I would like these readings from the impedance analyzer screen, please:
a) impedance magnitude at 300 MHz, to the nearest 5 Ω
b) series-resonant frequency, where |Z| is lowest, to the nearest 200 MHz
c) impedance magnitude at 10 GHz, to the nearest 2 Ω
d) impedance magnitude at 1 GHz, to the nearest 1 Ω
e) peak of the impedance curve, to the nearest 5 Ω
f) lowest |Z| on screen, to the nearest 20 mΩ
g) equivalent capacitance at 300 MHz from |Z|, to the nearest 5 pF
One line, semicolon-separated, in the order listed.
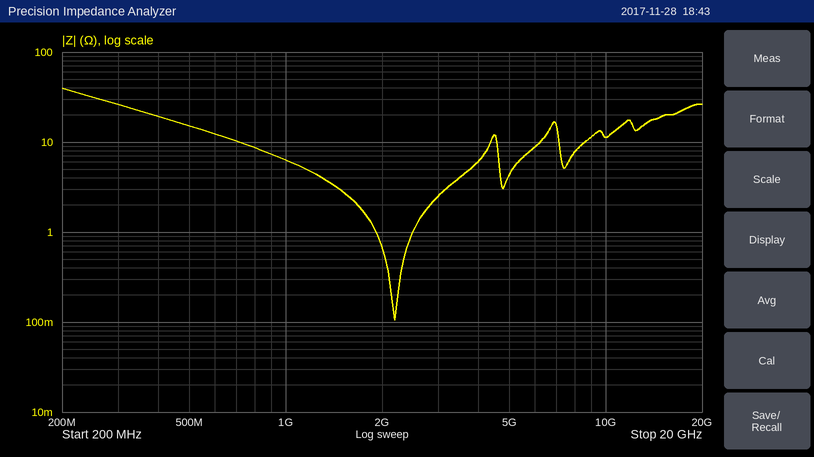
25 Ω; 2.2 GHz; 12 Ω; 6 Ω; 40 Ω; 100 mΩ; 20 pF
